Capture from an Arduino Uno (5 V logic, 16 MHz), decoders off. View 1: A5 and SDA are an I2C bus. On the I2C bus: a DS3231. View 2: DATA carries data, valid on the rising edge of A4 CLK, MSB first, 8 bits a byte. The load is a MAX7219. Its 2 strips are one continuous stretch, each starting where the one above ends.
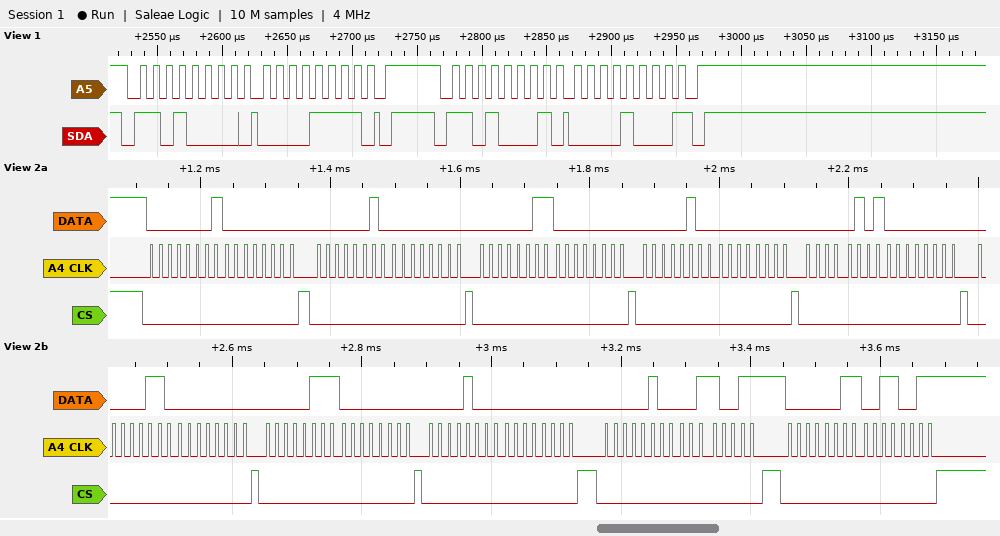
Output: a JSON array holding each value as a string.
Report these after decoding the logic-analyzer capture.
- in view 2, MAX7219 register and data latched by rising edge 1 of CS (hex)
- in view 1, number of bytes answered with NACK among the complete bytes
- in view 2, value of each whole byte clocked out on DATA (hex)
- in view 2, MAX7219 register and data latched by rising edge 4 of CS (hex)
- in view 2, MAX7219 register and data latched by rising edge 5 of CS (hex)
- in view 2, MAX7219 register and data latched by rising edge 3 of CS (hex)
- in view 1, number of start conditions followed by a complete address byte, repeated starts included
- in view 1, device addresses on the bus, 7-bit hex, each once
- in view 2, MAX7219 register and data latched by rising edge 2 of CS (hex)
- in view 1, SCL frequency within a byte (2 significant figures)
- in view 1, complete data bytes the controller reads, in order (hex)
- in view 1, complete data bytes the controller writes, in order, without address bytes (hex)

["register 0x1, data 0x00", "1", "0x01 0x00 0x02 0x00 0x03 0x00 0x04 0x00 0x05 0x00 0x06 0x00 0x07 0x00 0x08 0x00 0x04 0x33 0x03 0x33", "register 0x4, data 0x00", "register 0x5, data 0x00", "register 0x3, data 0x00", "2", "0x68", "register 0x2, data 0x00", "100 kHz", "08", "0F"]
